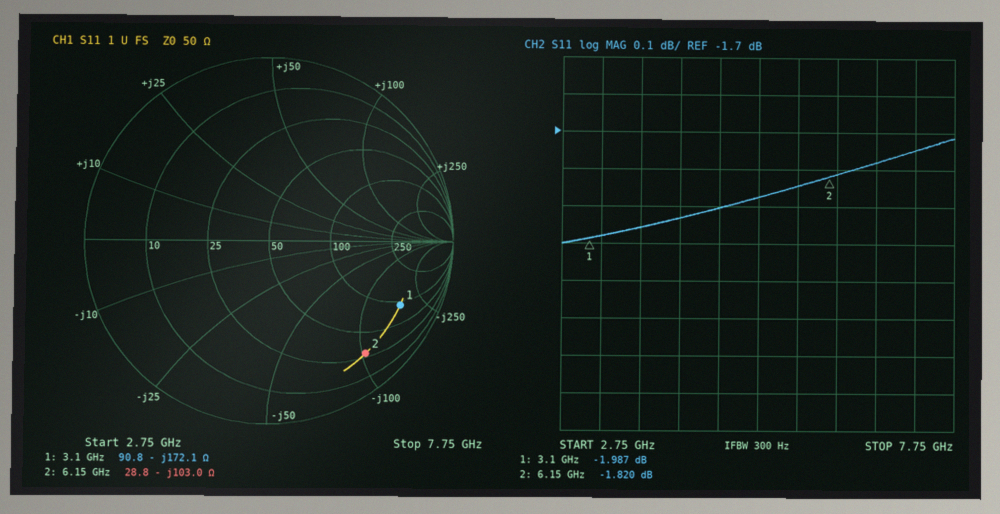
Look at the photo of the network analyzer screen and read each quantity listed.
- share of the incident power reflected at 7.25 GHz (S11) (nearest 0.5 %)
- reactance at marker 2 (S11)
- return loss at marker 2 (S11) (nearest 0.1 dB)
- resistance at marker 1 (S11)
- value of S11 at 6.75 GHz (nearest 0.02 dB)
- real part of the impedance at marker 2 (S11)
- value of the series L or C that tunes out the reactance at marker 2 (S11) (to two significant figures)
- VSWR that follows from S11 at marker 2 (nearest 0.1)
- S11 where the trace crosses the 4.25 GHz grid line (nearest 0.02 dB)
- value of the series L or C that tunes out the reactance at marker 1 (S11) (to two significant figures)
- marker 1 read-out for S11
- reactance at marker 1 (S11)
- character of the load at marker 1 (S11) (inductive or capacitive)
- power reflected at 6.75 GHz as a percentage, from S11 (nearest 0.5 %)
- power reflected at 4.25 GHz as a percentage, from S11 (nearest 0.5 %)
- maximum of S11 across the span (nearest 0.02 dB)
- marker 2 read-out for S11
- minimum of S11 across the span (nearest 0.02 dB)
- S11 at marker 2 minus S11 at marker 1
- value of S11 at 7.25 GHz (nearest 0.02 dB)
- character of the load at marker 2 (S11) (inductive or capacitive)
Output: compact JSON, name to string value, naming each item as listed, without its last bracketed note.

{"share of the incident power reflected at 7.25 GHz (S11)": "67.0 %", "reactance at marker 2": "-103.0 Ω", "return loss at marker 2 (S11)": "1.8 dB", "resistance at marker 1": "90.8 Ω", "value of S11 at 6.75 GHz": "-1.78 dB", "real part of the impedance at marker 2": "28.8 Ω", "value of the series L or C that tunes out the reactance at marker 2 (S11)": "2.7 nH", "VSWR that follows from S11 at marker 2": "9.6", "S11 where the trace crosses the 4.25 GHz grid line": "-1.94 dB", "value of the series L or C that tunes out the reactance at marker 1 (S11)": "8.8 nH", "marker 1 read-out for S11": "-1.987 dB", "reactance at marker 1": "-172.1 Ω", "character of the load at marker 1 (S11)": "capacitive", "power reflected at 6.75 GHz as a percentage, from S11": "66.5 %", "power reflected at 4.25 GHz as a percentage, from S11": "64.0 %", "maximum of S11 across the span": "-1.72 dB", "marker 2 read-out for S11": "-1.820 dB", "minimum of S11 across the span": "-2.00 dB", "S11 at marker 2 minus S11 at marker 1": "0.167 dB", "value of S11 at 7.25 GHz": "-1.74 dB", "character of the load at marker 2 (S11)": "capacitive"}
